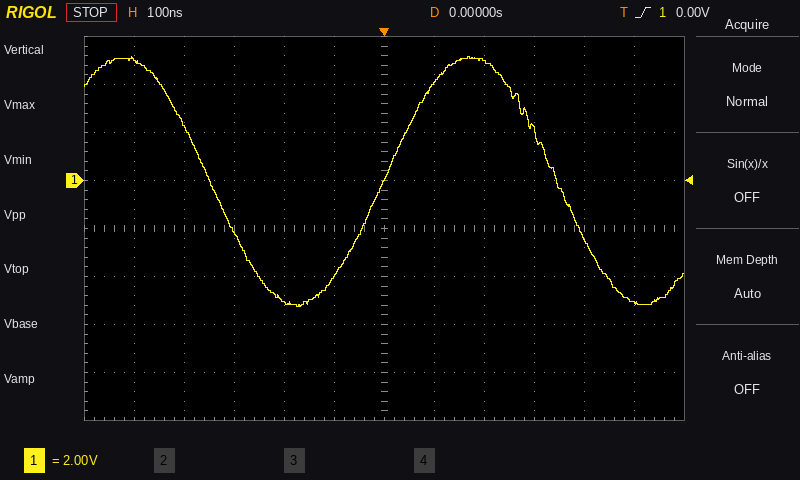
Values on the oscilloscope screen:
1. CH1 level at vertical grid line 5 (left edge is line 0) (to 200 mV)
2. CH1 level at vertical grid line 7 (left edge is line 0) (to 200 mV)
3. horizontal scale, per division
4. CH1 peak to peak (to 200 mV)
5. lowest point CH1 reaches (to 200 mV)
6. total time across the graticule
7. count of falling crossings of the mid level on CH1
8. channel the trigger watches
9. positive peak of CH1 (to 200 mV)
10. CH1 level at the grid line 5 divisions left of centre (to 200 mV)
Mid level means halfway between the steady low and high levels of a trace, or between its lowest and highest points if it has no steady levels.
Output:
-4.0 V
4.0 V
100 ns
10.4 V
-5.2 V
1.2 µs
2
CH1
5.2 V
5.0 V
